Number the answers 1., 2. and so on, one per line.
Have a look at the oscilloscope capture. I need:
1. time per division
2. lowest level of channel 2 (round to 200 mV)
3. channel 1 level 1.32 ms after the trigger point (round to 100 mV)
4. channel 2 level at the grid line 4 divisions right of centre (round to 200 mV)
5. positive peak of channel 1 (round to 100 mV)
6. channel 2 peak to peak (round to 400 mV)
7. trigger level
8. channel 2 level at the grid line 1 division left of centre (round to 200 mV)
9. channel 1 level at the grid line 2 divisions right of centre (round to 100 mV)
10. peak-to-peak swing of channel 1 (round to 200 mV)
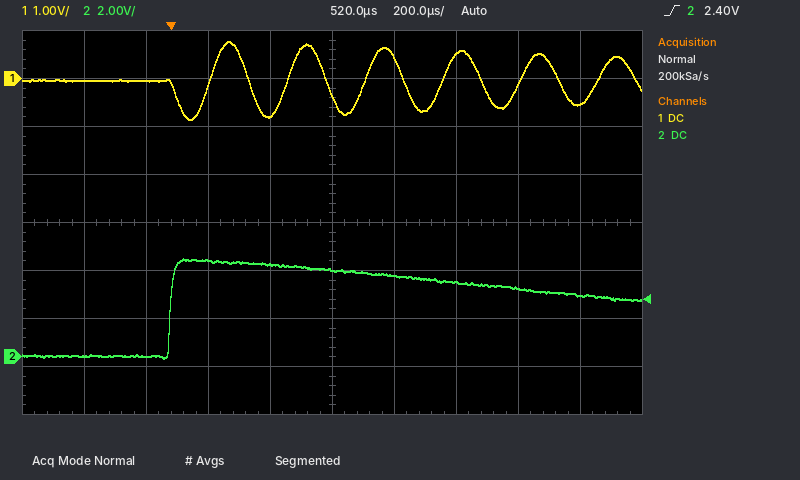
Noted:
1. 200 µs
2. 0.0 V
3. -500 mV
4. 2.6 V
5. 800 mV
6. 4.0 V
7. 2.40 V
8. 3.8 V
9. 500 mV
10. 1.6 V
